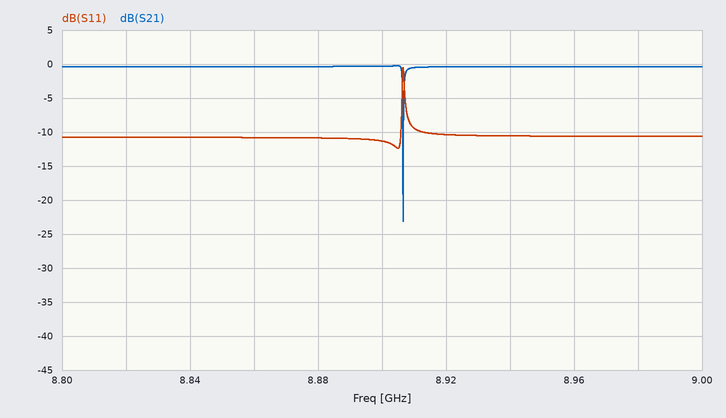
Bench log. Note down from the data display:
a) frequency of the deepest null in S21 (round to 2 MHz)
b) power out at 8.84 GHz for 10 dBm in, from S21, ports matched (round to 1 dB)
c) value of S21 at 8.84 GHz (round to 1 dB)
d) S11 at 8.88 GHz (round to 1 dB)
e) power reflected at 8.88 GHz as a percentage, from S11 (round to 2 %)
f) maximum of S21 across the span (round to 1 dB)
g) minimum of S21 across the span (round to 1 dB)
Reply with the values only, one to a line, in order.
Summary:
8.906 GHz
10 dBm
0 dB
-11 dB
8 %
0 dB
-23 dB
